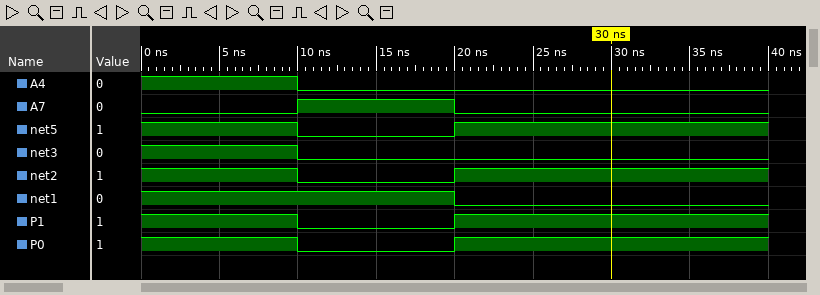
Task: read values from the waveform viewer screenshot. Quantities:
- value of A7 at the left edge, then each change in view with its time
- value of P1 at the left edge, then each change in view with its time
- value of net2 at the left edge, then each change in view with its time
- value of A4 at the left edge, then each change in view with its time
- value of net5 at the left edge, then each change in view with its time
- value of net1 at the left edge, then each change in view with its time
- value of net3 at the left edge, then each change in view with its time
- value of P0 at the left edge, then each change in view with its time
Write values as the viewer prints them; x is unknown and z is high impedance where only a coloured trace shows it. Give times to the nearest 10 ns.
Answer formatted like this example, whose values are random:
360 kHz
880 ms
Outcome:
0, 1 at 10 ns, 0 at 20 ns
1, 0 at 10 ns, 1 at 20 ns
1, 0 at 10 ns, 1 at 20 ns
1, 0 at 10 ns
1, 0 at 10 ns, 1 at 20 ns
1, 0 at 20 ns
1, 0 at 10 ns
1, 0 at 10 ns, 1 at 20 ns
